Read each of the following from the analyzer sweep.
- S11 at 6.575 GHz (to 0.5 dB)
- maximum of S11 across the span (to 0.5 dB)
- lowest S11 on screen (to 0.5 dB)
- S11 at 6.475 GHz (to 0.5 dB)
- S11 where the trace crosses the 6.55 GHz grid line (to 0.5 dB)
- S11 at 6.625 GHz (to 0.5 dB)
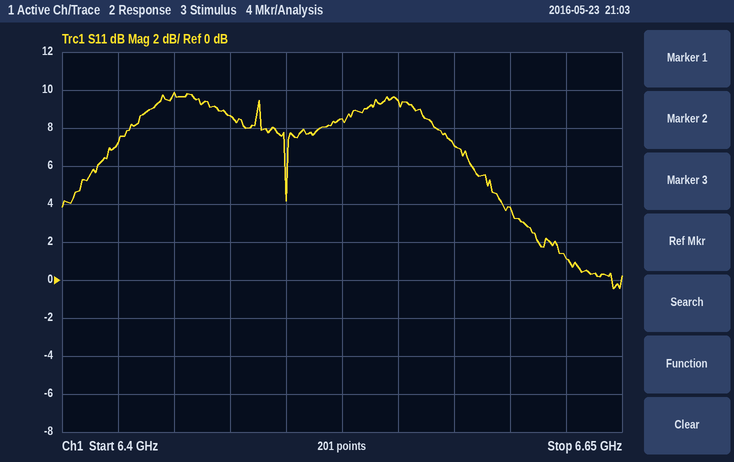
7.0 dB
10.0 dB
-0.5 dB
8.5 dB
9.5 dB
1.0 dB
